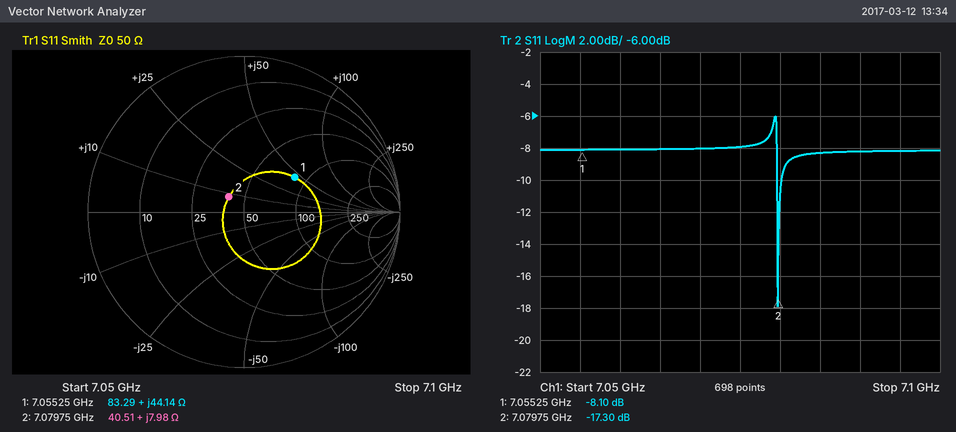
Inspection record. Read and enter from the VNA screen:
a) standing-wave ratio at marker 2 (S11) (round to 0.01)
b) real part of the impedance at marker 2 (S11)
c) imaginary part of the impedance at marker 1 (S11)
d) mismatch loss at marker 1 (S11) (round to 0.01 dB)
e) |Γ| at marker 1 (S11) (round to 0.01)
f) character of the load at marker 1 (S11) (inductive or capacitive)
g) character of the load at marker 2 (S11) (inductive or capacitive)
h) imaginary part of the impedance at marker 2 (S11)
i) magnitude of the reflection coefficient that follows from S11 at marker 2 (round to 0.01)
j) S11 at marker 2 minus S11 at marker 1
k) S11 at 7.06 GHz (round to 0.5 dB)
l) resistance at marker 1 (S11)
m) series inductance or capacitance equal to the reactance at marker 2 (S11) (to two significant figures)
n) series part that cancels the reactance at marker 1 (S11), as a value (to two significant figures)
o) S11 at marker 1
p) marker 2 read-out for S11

1.32
40.51 Ω
+44.14 Ω
0.73 dB
0.39
inductive
inductive
+7.98 Ω
0.14
-9.20 dB
-8.0 dB
83.29 Ω
180 pH
510 fF
-8.10 dB
-17.30 dB
